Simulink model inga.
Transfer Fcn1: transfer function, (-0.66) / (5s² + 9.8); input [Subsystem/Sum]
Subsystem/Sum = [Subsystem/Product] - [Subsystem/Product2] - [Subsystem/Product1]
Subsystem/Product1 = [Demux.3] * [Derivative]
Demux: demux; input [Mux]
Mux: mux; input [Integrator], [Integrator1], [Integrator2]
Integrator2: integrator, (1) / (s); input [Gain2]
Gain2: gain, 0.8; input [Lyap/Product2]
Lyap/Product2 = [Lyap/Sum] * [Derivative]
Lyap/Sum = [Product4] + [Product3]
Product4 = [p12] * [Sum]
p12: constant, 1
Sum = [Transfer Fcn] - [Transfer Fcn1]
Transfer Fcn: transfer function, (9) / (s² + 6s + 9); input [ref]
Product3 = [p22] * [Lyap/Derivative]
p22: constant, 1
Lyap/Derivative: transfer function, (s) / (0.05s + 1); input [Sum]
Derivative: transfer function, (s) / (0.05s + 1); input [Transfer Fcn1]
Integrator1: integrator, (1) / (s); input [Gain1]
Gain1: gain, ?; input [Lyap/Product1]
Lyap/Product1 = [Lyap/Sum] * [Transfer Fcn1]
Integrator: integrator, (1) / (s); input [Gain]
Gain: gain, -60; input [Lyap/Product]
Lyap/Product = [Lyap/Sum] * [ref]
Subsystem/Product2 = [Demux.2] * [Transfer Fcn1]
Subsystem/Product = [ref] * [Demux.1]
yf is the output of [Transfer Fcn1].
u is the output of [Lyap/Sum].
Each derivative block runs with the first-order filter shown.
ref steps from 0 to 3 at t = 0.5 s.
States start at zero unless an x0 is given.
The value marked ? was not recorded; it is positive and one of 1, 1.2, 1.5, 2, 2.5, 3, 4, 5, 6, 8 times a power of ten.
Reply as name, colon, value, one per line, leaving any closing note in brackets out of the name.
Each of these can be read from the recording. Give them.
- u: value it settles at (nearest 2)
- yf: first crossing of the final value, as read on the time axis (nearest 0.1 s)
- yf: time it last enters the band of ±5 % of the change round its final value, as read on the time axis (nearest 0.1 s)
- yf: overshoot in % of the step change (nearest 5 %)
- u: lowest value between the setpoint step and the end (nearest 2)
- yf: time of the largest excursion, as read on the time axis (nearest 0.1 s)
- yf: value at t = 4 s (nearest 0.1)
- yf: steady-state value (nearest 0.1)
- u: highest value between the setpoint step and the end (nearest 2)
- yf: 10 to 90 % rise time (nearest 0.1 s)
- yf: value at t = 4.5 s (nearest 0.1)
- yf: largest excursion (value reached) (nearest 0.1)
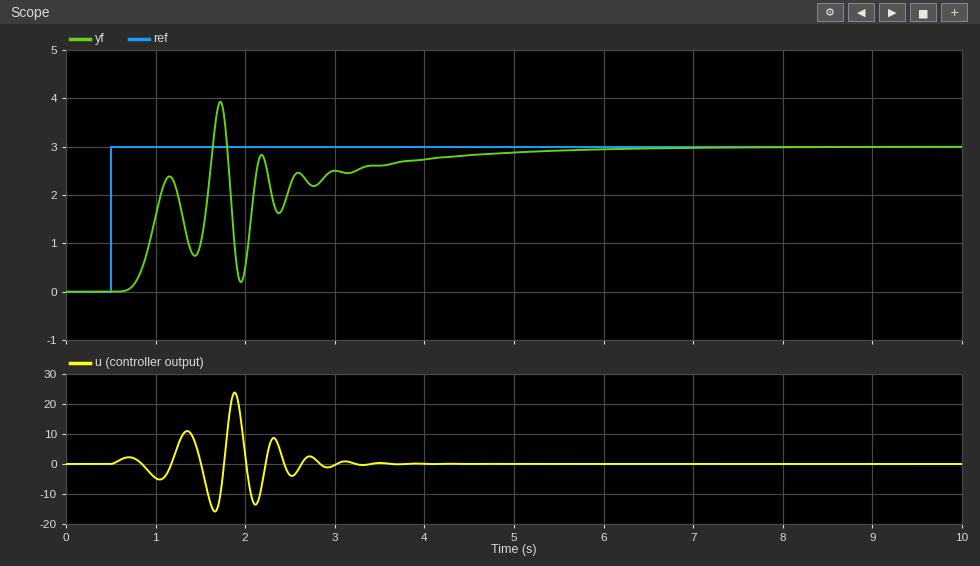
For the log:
u: value it settles at: 0
yf: first crossing of the final value, as read on the time axis: 1.6 s
yf: time it last enters the band of ±5 % of the change round its final value, as read on the time axis: 4.7 s
yf: overshoot in % of the step change: 30 %
u: lowest value between the setpoint step and the end: -16
yf: time of the largest excursion, as read on the time axis: 1.7 s
yf: value at t = 4 s: 2.7
yf: steady-state value: 3.0
u: highest value between the setpoint step and the end: 24
yf: 10 to 90 % rise time: 0.8 s
yf: value at t = 4.5 s: 2.8
yf: largest excursion (value reached): 3.9
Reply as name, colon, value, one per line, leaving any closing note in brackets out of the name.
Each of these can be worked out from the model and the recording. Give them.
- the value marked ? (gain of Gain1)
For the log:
the value marked ?: 80
